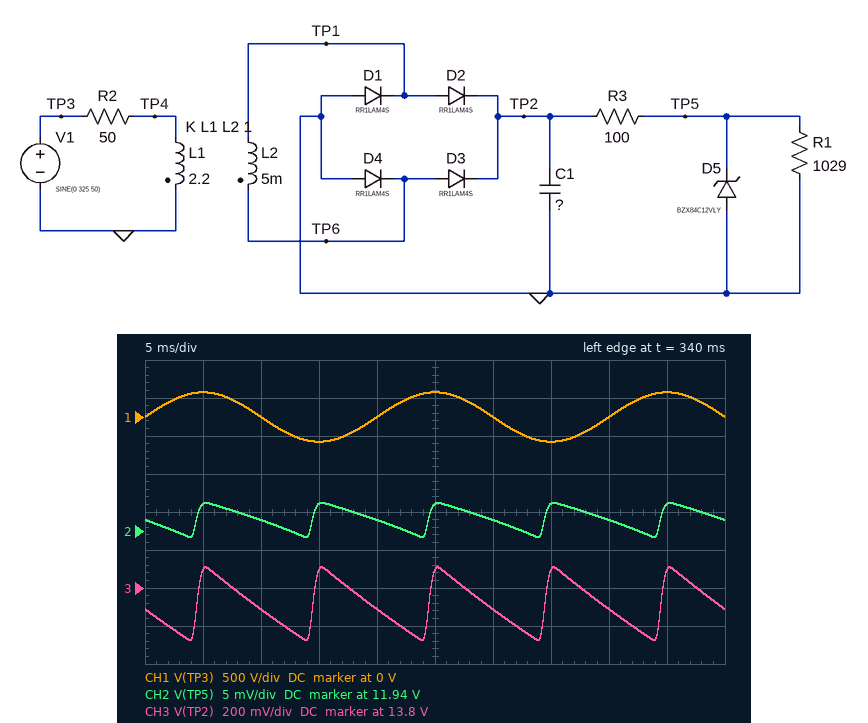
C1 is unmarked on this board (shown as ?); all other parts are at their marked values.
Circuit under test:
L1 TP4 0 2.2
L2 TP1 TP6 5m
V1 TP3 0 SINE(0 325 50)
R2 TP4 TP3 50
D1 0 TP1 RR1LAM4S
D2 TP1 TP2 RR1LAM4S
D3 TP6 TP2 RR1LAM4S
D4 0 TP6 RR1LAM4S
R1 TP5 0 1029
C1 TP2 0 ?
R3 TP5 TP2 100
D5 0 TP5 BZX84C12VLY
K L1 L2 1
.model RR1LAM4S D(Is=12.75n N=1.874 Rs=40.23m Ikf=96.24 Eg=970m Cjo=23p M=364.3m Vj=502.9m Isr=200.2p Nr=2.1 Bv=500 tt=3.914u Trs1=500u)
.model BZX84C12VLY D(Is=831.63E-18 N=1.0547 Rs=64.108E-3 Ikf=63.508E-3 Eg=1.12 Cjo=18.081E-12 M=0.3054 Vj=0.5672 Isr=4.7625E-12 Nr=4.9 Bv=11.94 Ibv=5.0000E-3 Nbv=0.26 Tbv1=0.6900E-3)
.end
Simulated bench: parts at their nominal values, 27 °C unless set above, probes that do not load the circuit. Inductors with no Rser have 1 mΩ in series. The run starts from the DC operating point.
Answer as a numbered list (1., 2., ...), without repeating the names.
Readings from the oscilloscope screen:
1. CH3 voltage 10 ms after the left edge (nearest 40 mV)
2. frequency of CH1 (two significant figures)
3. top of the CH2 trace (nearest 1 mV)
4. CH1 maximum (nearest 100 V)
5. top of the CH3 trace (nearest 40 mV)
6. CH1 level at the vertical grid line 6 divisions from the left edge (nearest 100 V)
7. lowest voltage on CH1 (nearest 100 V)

1. 13.68 V
2. 50 Hz
3. 11.944 V
4. 300 V
5. 13.92 V
6. 0 V
7. -300 V
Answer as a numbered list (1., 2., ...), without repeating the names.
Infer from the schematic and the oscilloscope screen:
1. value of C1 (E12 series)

1. 390 µF
